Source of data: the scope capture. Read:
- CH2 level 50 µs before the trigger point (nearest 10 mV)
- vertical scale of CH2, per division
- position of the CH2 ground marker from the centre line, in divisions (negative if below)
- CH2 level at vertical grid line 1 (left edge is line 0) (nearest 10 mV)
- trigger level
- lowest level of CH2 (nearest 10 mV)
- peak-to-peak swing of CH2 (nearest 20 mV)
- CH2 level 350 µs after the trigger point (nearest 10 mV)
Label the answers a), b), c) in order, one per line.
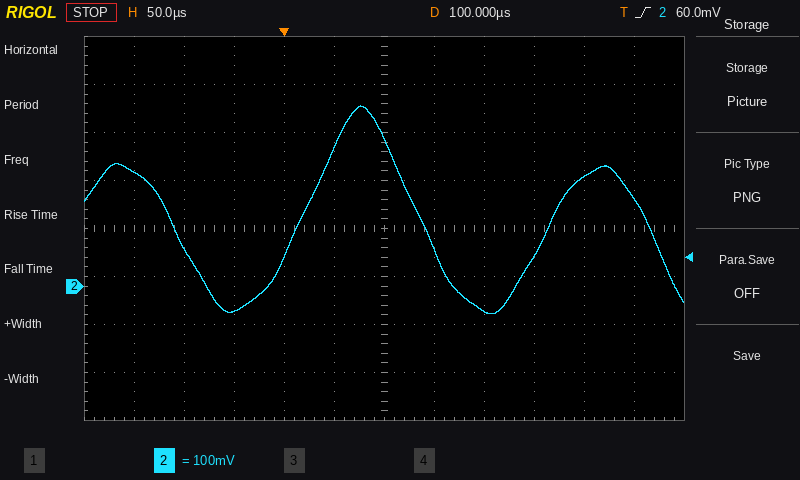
a) -50 mV
b) 100 mV
c) -1.2 div
d) 240 mV
e) 60.0 mV
f) -60 mV
g) 440 mV
h) 180 mV
